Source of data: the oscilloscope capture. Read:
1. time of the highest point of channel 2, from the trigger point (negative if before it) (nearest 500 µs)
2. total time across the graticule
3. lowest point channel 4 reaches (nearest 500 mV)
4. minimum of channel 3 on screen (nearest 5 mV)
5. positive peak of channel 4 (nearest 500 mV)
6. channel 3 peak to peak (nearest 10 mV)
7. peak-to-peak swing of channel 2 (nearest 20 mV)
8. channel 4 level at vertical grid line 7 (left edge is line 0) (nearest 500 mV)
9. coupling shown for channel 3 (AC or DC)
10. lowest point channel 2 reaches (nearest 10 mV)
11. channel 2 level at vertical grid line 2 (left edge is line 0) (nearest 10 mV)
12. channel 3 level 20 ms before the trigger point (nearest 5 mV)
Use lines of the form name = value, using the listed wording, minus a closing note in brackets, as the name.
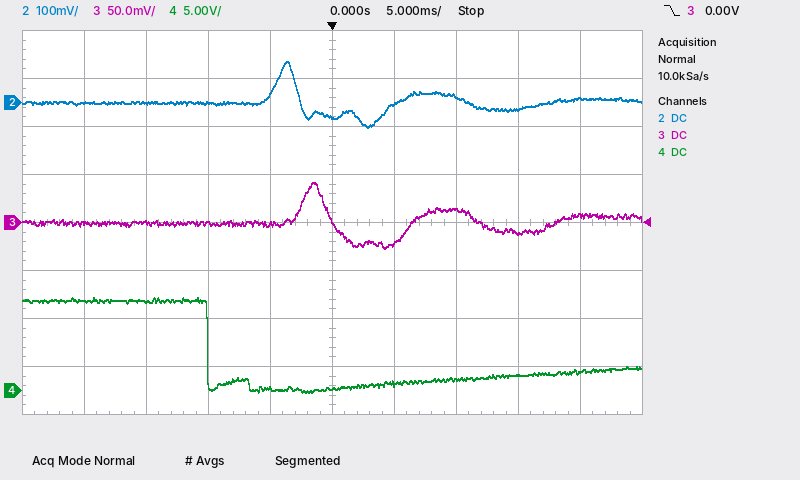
time of the highest point of channel 2, from the trigger point (negative if before it) = -3.5 ms
total time across the graticule = 50 ms
lowest point channel 4 reaches = 0.0 V
minimum of channel 3 on screen = -25 mV
positive peak of channel 4 = 9.5 V
channel 3 peak to peak = 70 mV
peak-to-peak swing of channel 2 = 140 mV
channel 4 level at vertical grid line 7 (left edge is line 0) = 1.0 V
coupling shown for channel 3 = DC
lowest point channel 2 reaches = -50 mV
channel 2 level at vertical grid line 2 (left edge is line 0) = 0 mV
channel 3 level 20 ms before the trigger point = 0 mV
